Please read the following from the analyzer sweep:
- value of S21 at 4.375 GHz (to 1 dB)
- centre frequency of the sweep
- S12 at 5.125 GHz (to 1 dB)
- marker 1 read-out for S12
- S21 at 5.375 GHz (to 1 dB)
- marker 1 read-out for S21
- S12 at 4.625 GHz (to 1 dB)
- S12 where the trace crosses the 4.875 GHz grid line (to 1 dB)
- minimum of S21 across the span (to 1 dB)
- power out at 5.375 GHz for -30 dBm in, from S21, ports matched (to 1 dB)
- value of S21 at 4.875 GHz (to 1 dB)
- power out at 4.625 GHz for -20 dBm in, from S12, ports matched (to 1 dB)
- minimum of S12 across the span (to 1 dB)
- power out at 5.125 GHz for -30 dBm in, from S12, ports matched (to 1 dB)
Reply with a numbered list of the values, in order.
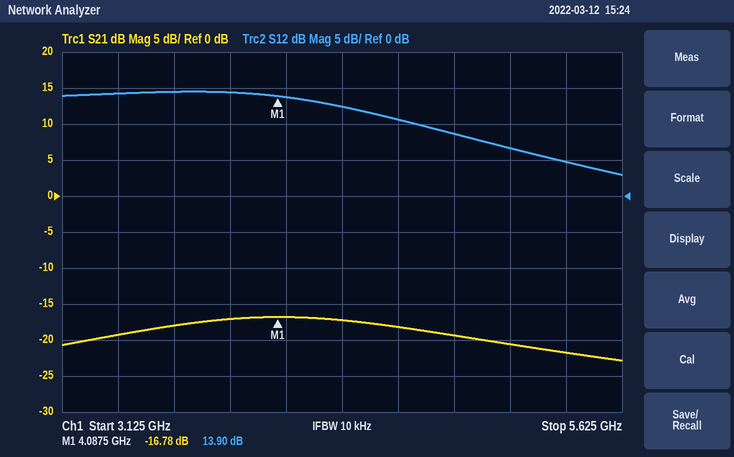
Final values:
1. -17 dB
2. 4.375 GHz
3. 7 dB
4. 13.90 dB
5. -22 dB
6. -16.78 dB
7. 11 dB
8. 9 dB
9. -23 dB
10. -52 dBm
11. -19 dB
12. -9 dBm
13. 3 dB
14. -23 dBm
